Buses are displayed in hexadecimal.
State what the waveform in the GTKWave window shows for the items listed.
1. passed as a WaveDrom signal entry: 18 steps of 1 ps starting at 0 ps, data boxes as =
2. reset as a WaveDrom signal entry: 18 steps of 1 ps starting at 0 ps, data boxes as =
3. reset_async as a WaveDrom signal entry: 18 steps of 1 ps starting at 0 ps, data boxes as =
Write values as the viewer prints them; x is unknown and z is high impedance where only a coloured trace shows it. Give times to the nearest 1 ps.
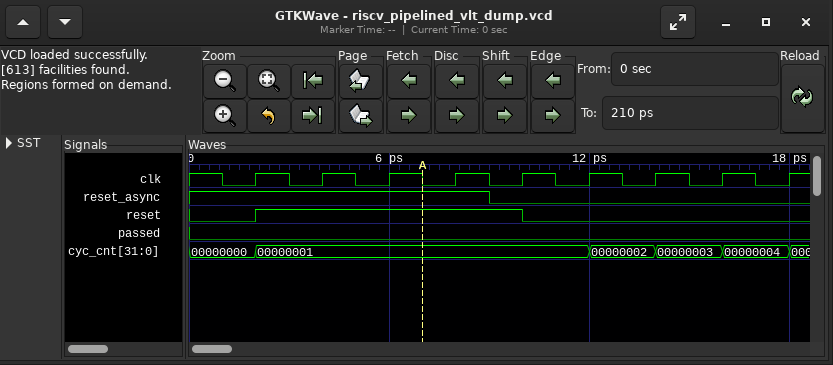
{name: 'passed', wave: '0.................'}
{name: 'reset', wave: '0.1.......0.......'}
{name: 'reset_async', wave: '1........0........'}
